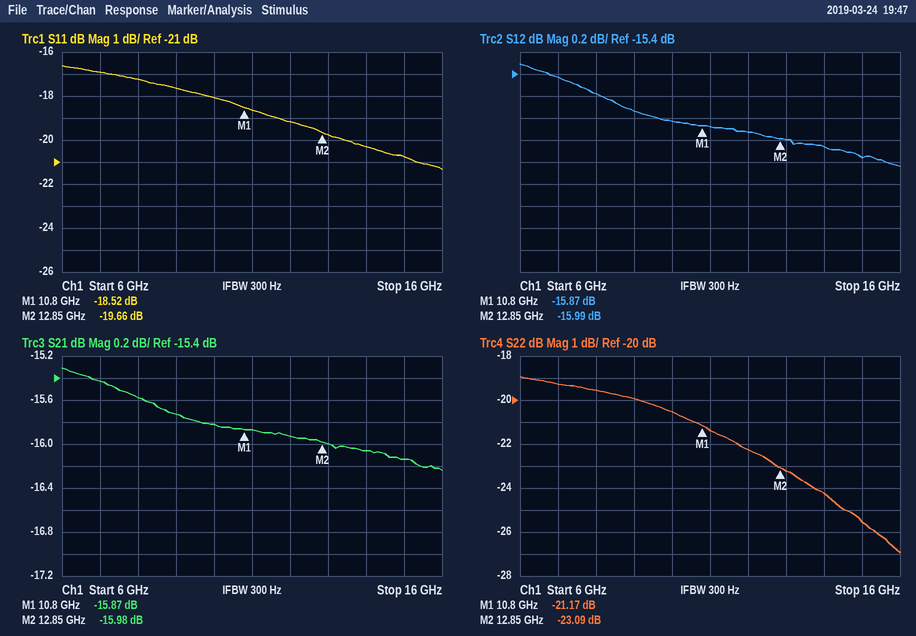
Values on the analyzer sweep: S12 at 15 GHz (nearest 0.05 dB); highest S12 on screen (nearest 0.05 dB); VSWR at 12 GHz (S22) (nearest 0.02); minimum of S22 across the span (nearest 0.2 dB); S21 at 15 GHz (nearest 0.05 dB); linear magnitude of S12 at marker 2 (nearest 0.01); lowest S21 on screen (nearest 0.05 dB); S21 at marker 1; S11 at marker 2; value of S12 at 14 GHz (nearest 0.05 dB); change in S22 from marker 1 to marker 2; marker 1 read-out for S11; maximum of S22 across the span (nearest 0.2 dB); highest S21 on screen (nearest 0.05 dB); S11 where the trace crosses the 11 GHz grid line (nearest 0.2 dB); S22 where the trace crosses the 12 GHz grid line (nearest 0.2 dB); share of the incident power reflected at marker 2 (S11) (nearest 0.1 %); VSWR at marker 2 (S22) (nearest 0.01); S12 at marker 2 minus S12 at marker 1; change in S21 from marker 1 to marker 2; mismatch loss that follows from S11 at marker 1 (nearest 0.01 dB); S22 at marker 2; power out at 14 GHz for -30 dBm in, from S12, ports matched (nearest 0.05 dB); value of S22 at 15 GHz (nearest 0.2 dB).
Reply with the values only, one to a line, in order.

-16.15 dB
-15.30 dB
1.16
-27.0 dB
-16.15 dB
0.16
-16.25 dB
-15.87 dB
-19.66 dB
-16.05 dB
-1.92 dB
-18.52 dB
-19.0 dB
-15.30 dB
-18.6 dB
-22.2 dB
1.1 %
1.15
-0.12 dB
-0.11 dB
0.06 dB
-23.09 dB
-46.05 dBm
-25.6 dB
